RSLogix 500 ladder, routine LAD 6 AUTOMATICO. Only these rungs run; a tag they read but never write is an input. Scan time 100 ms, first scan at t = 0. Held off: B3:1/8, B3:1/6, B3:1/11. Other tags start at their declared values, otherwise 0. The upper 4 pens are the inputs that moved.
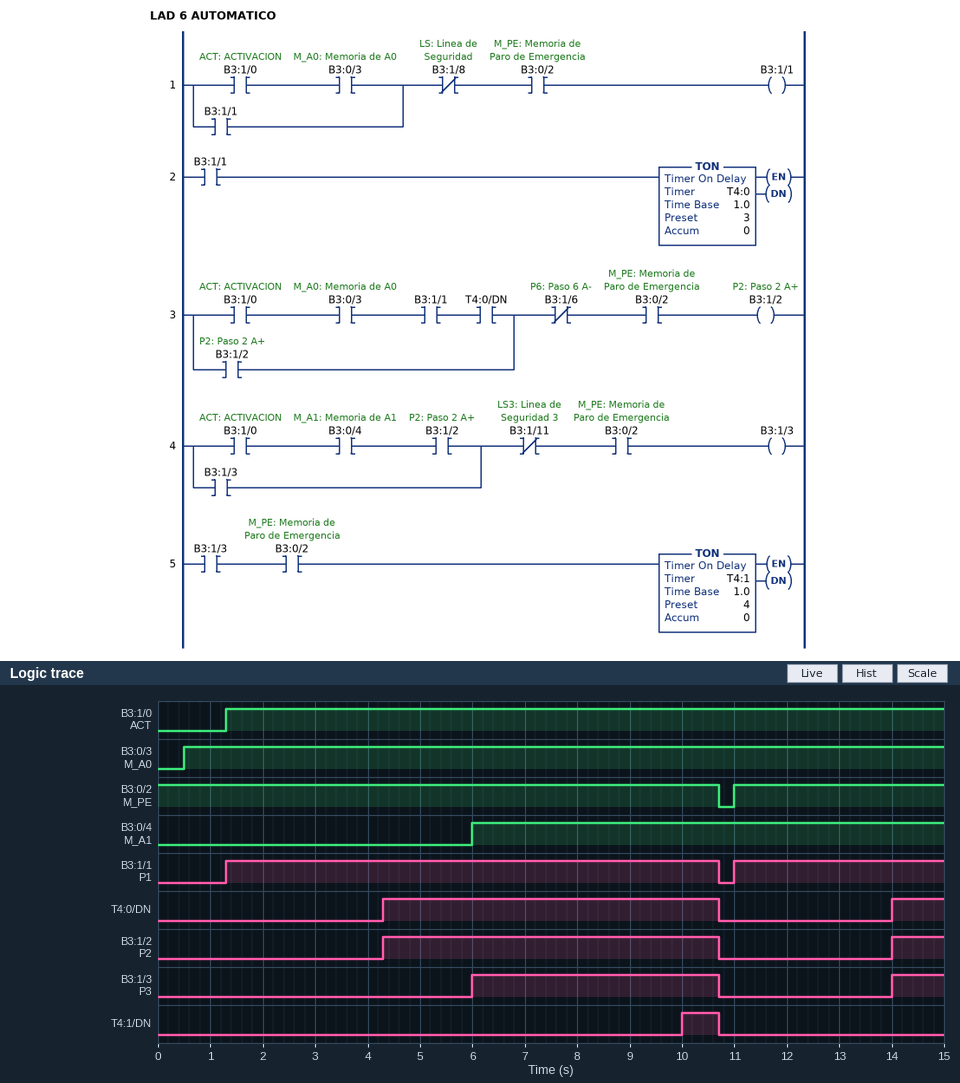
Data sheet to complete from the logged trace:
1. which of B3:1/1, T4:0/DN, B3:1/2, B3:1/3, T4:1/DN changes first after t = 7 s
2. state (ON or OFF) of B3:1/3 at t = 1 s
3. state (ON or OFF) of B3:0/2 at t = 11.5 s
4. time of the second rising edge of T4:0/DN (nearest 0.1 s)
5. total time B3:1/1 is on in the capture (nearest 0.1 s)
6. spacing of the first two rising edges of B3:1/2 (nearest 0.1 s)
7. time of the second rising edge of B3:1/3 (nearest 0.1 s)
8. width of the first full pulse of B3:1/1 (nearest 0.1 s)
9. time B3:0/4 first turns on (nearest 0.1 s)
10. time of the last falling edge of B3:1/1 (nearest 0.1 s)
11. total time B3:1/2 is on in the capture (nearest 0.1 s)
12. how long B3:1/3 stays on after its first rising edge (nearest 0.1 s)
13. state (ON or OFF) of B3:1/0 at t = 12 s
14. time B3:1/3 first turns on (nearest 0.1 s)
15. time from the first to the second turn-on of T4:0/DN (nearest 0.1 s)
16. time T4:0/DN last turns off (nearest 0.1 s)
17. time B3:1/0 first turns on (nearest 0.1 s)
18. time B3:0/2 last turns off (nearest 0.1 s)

T4:1/DN
OFF
ON
14.0 s
13.4 s
9.7 s
14.0 s
9.4 s
6.0 s
10.7 s
7.4 s
4.7 s
ON
6.0 s
9.7 s
10.7 s
1.3 s
10.7 s
